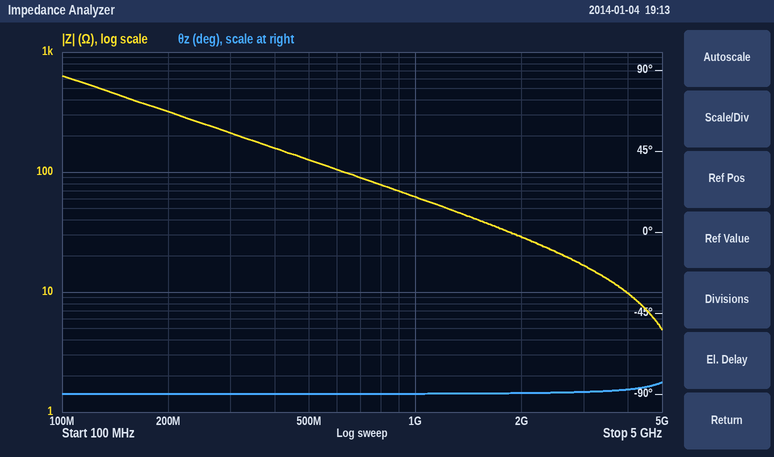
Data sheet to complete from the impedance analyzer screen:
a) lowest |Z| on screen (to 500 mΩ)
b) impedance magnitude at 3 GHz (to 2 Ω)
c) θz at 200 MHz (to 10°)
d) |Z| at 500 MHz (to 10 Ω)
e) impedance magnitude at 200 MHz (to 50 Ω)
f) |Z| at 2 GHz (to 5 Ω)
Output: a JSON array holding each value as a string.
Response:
["5.0 Ω", "16 Ω", "-90°", "130 Ω", "300 Ω", "30 Ω"]
